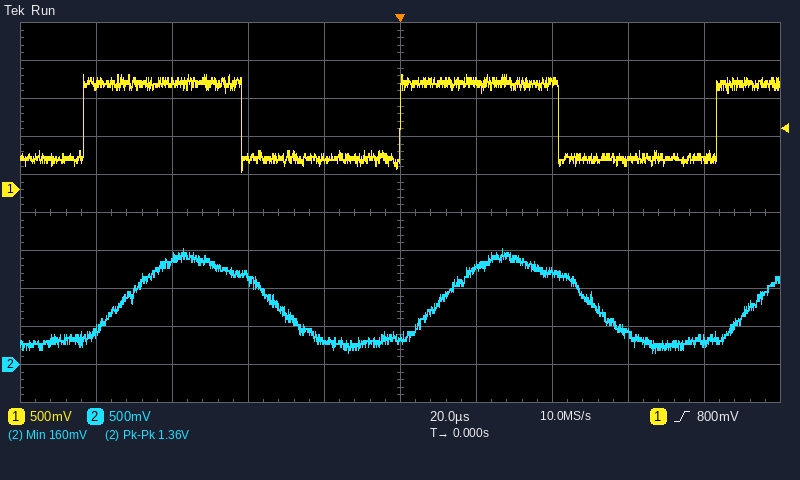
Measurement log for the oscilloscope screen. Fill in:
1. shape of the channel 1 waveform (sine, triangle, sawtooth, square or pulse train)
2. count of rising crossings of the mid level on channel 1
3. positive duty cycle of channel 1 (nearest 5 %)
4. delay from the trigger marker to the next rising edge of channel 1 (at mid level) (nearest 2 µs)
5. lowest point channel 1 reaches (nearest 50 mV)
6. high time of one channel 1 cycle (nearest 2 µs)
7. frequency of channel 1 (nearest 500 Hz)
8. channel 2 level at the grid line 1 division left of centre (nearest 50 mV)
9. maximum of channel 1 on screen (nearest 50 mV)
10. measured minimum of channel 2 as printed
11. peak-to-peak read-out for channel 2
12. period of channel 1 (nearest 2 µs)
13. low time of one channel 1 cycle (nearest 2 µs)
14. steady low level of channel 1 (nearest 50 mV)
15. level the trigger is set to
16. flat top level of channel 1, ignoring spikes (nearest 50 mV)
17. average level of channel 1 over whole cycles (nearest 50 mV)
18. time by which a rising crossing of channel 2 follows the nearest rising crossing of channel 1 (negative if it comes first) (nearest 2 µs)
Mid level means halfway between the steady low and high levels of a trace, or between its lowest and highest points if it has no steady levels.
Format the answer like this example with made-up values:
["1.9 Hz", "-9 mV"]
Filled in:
["square", "3", "50 %", "84 µs", "250 mV", "42 µs", "12.0 kHz", "300 mV", "1.50 V", "160 mV", "1.36 V", "84 µs", "42 µs", "400 mV", "800 mV", "1.40 V", "900 mV", "+10 µs"]
